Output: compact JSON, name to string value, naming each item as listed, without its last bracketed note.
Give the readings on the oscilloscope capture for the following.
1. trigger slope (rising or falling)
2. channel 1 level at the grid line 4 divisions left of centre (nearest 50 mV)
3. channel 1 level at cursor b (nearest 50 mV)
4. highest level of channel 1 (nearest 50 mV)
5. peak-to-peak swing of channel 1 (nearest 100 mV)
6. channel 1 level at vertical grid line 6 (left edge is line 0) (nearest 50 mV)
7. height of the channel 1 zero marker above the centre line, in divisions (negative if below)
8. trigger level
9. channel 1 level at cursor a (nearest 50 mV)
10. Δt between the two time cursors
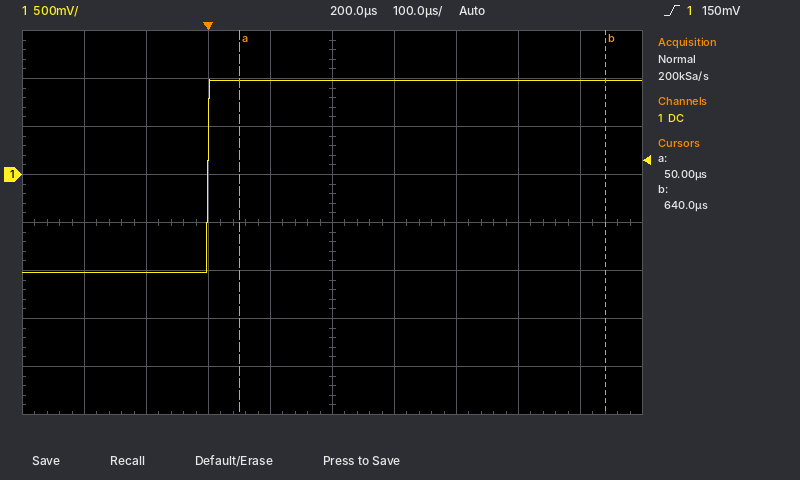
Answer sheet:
{"trigger slope": "rising", "channel 1 level at the grid line 4 divisions left of centre": "-1.00 V", "channel 1 level at cursor b": "1.00 V", "highest level of channel 1": "1.00 V", "peak-to-peak swing of channel 1": "2.00 V", "channel 1 level at vertical grid line 6 (left edge is line 0)": "1.00 V", "height of the channel 1 zero marker above the centre line, in divisions": "+1.0 div", "trigger level": "150 mV", "channel 1 level at cursor a": "1.00 V", "Δt between the two time cursors": "590 µs"}
